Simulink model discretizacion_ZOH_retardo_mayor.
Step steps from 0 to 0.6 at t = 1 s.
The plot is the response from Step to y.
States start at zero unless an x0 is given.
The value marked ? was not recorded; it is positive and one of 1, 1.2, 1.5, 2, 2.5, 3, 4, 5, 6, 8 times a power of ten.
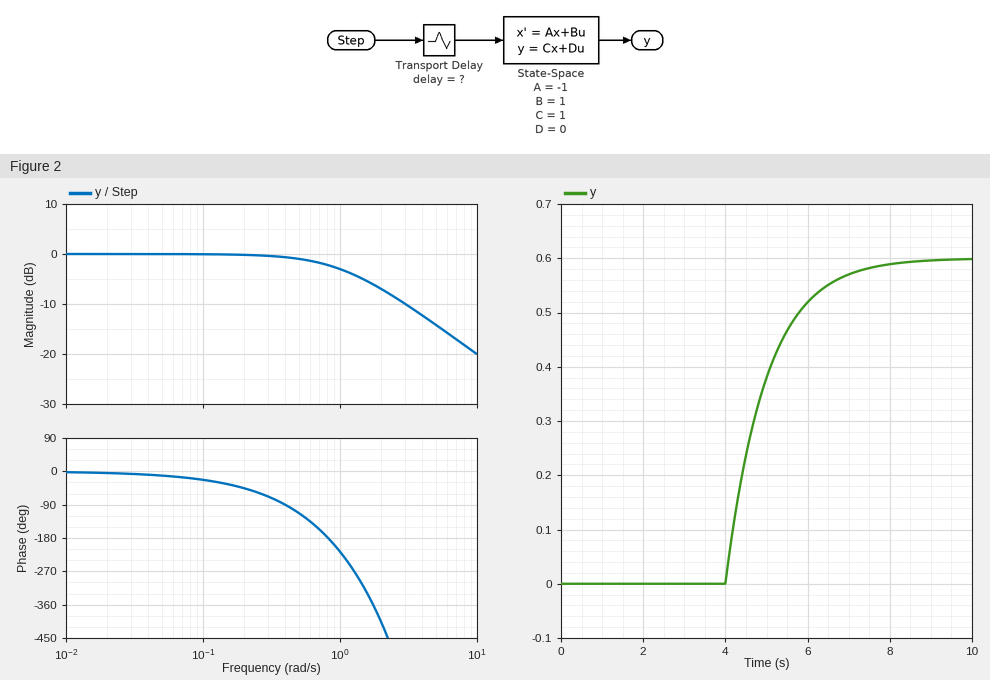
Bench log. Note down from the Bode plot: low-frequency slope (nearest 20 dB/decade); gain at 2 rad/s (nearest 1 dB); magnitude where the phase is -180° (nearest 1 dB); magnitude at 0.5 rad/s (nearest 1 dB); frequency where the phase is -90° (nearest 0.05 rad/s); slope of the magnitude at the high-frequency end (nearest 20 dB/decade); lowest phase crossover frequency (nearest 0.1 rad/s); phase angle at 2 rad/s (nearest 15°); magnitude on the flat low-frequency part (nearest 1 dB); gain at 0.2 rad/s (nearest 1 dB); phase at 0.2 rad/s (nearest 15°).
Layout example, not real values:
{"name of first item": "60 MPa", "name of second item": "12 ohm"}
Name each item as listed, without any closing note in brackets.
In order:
{"low-frequency slope": "0 dB/decade", "gain at 2 rad/s": "-7 dB", "magnitude where the phase is -180°": "-2 dB", "magnitude at 0.5 rad/s": "-1 dB", "frequency where the phase is -90°": "0.40 rad/s", "slope of the magnitude at the high-frequency end": "-20 dB/decade", "lowest phase crossover frequency": "0.8 rad/s", "phase angle at 2 rad/s": "-405°", "magnitude on the flat low-frequency part": "0 dB", "gain at 0.2 rad/s": "0 dB", "phase at 0.2 rad/s": "-45°"}
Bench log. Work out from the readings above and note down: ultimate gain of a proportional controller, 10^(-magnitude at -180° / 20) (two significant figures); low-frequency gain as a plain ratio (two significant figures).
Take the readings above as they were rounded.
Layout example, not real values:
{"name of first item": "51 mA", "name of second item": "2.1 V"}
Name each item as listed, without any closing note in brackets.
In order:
{"ultimate gain of a proportional controller, 10^(-magnitude at -180° / 20)": "1.3", "low-frequency gain as a plain ratio": "1.0"}
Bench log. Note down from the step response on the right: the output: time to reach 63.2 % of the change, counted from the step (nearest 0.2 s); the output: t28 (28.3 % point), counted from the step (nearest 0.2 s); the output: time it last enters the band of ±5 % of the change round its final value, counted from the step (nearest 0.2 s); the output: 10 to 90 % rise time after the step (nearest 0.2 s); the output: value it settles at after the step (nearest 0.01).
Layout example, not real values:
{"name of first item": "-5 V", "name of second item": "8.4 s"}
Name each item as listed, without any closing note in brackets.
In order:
{"the output: time to reach 63.2 % of the change, counted from the step": "4.0 s", "the output: t28 (28.3 % point), counted from the step": "3.4 s", "the output: time it last enters the band of ±5 % of the change round its final value, counted from the step": "6.0 s", "the output: 10 to 90 % rise time after the step": "2.2 s", "the output: value it settles at after the step": "0.60"}
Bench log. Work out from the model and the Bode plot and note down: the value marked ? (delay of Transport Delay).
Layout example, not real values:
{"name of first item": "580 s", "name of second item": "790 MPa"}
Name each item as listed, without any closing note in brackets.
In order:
{"the value marked ?": "3"}
